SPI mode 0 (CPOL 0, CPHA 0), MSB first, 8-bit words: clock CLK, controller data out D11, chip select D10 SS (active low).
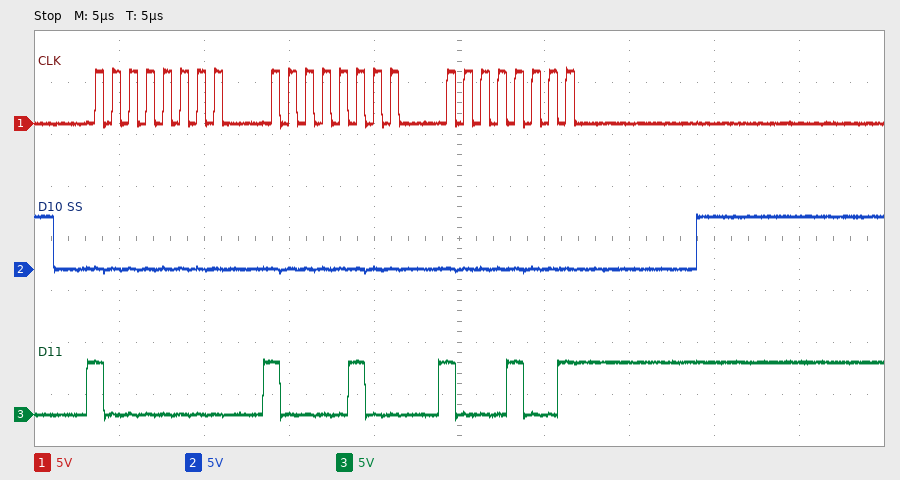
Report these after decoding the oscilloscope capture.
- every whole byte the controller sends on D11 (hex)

0x80 0x84 0x89
